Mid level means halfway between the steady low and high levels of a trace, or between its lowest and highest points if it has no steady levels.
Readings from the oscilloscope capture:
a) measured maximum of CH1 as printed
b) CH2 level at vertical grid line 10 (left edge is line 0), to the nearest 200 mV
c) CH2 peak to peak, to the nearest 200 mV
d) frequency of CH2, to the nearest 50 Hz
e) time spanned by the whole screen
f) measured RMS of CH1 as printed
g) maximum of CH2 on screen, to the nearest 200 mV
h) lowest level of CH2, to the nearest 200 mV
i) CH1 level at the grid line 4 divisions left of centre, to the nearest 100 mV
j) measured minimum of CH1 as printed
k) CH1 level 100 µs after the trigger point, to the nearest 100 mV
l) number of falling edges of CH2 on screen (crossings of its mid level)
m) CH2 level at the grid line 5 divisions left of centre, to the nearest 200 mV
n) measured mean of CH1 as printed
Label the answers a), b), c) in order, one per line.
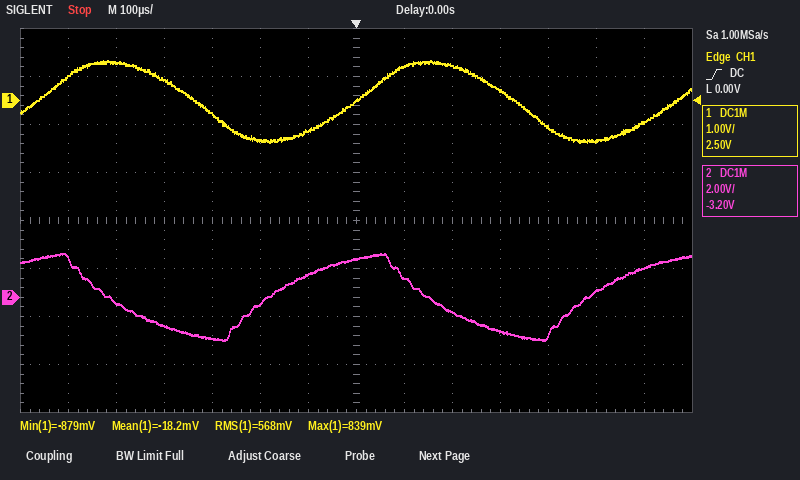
a) 839 mV
b) -1.4 V
c) 3.6 V
d) 1.50 kHz
e) 1.4 ms
f) 568 mV
g) 1.8 V
h) -1.8 V
i) 400 mV
j) -879 mV
k) 700 mV
l) 2
m) -200 mV
n) -18.2 mV
